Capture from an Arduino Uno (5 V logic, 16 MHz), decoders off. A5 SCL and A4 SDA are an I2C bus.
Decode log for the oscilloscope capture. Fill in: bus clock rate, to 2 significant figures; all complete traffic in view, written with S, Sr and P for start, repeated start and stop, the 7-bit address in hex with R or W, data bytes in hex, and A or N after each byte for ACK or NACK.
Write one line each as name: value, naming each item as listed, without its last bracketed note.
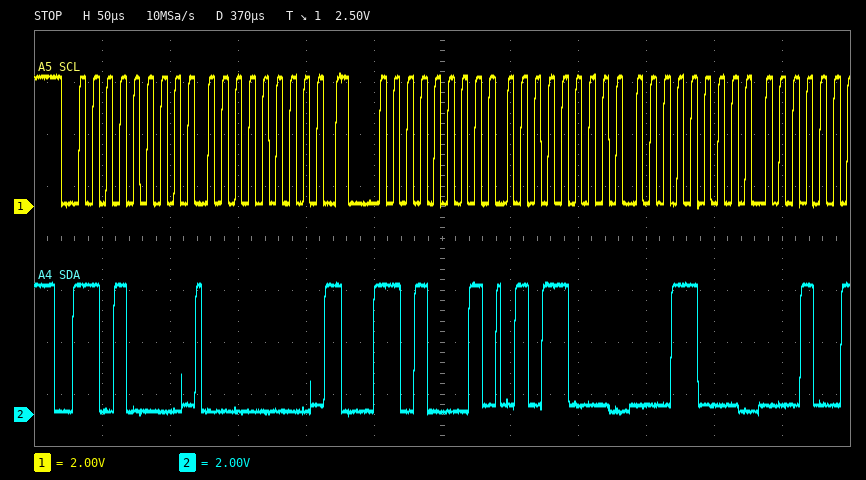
bus clock rate, to 2 significant figures: 100 kHz
all complete traffic in view, written with S, Sr and P for start, repeated start and stop, the 7-bit address in hex with R or W, data bytes in hex, and A or N after each byte for ACK or NACK: S 68W A 00 A Sr 68R A 58 A 18 A
